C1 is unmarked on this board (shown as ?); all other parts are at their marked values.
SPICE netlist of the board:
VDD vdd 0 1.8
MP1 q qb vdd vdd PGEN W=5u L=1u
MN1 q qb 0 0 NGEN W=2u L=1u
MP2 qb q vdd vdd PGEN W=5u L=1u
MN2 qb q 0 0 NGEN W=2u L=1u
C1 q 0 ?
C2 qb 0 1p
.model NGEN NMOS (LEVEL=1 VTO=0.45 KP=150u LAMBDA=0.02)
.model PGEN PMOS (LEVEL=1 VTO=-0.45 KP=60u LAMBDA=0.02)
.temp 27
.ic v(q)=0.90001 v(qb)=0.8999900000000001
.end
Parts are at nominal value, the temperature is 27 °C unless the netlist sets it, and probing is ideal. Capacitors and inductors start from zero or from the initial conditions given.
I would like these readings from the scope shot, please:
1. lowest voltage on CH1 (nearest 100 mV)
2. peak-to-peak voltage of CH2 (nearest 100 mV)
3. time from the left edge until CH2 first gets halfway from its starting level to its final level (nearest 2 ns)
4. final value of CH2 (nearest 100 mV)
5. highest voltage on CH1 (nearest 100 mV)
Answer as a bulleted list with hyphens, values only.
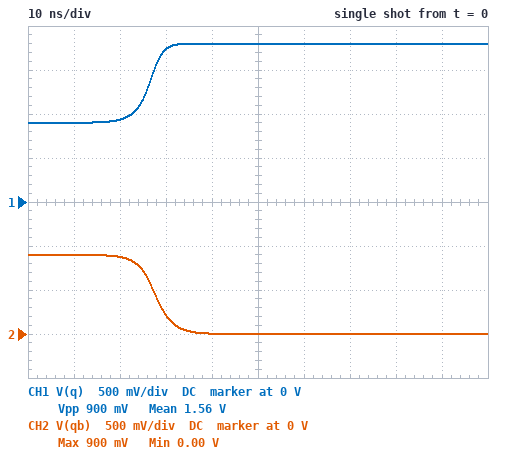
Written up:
- 900 mV
- 900 mV
- 28 ns
- 0 V
- 1.8 V
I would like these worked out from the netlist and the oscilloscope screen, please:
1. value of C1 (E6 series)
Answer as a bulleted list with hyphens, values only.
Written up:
- 470 fF
